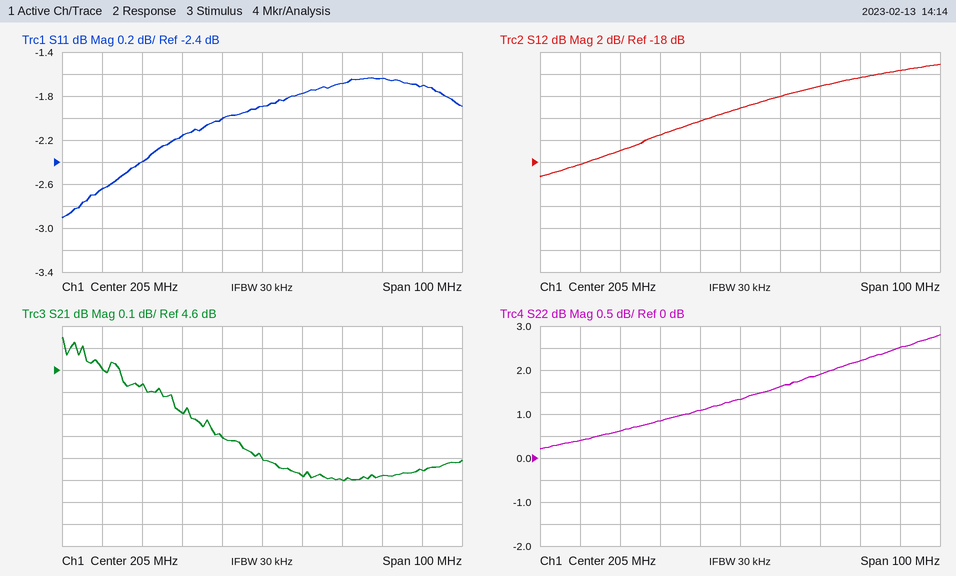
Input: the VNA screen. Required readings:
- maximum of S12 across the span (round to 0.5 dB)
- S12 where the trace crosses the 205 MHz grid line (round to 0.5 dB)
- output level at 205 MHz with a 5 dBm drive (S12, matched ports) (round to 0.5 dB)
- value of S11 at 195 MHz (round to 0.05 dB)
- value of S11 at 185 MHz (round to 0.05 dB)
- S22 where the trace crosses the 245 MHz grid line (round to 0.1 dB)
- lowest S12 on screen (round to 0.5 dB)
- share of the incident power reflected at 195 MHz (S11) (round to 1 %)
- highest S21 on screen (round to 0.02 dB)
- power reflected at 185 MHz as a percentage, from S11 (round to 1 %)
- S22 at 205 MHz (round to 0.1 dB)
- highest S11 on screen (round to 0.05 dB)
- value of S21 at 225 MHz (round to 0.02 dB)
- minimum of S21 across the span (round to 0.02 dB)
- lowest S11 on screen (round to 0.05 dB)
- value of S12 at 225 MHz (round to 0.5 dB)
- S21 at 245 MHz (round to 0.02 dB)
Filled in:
-9.0 dB
-13.0 dB
-8.0 dBm
-2.00 dB
-2.15 dB
2.5 dB
-19.5 dB
63 %
4.74 dB
61 %
1.3 dB
-1.65 dB
4.10 dB
4.10 dB
-2.90 dB
-11.0 dB
4.14 dB
